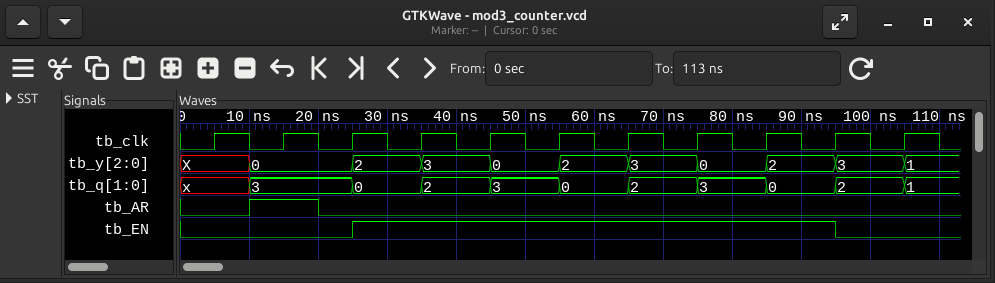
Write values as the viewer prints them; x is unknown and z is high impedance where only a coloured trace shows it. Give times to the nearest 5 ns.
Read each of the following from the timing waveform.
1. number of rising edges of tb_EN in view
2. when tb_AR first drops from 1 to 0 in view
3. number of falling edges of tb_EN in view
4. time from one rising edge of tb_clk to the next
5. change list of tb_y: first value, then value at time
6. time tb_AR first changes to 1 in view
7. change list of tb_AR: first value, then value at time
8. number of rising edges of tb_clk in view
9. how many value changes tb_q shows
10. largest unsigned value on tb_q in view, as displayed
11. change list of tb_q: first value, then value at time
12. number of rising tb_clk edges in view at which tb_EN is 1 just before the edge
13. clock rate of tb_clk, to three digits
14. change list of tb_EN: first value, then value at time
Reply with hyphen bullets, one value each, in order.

- 1
- 20 ns
- 1
- 10 ns
- X, 0 at 10 ns, 2 at 25 ns, 3 at 35 ns, 0 at 45 ns, 2 at 55 ns, 3 at 65 ns, 0 at 75 ns, 2 at 85 ns, 3 at 95 ns, 1 at 105 ns
- 10 ns
- 0, 1 at 10 ns, 0 at 20 ns
- 11
- 10
- 3
- x, 3 at 10 ns, 0 at 25 ns, 2 at 35 ns, 3 at 45 ns, 0 at 55 ns, 2 at 65 ns, 3 at 75 ns, 0 at 85 ns, 2 at 95 ns, 1 at 105 ns
- 7
- 100 MHz
- 0, 1 at 25 ns, 0 at 95 ns
